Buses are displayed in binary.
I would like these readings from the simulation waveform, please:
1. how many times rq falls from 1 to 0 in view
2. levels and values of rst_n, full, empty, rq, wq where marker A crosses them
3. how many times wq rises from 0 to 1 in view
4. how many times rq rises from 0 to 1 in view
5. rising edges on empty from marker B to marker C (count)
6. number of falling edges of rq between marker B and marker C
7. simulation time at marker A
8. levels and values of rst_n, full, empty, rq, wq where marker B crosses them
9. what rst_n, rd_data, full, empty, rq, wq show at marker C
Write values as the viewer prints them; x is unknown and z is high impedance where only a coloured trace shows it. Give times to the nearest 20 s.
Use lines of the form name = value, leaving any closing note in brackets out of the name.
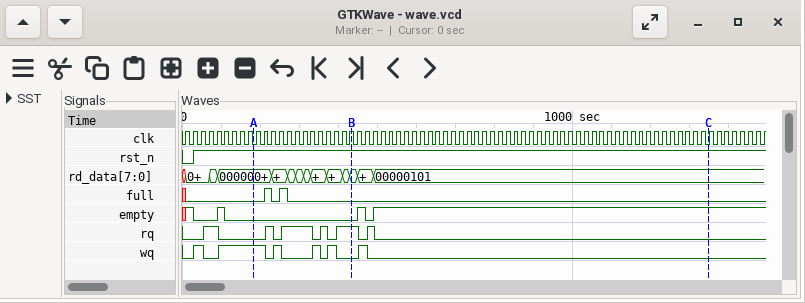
how many times rq falls from 1 to 0 in view = 6
levels and values of rst_n, full, empty, rq, wq where marker A crosses them = rst_n=1, full=0, empty=0, rq=0, wq=1
how many times wq rises from 0 to 1 in view = 6
how many times rq rises from 0 to 1 in view = 6
rising edges on empty from marker B to marker C = 2
number of falling edges of rq between marker B and marker C = 2
simulation time at marker A = 180 s
levels and values of rst_n, full, empty, rq, wq where marker B crosses them = rst_n=1, full=0, empty=0, rq=1, wq=0
what rst_n, rd_data, full, empty, rq, wq show at marker C = rst_n=1, rd_data=00000101, full=0, empty=1, rq=0, wq=0
